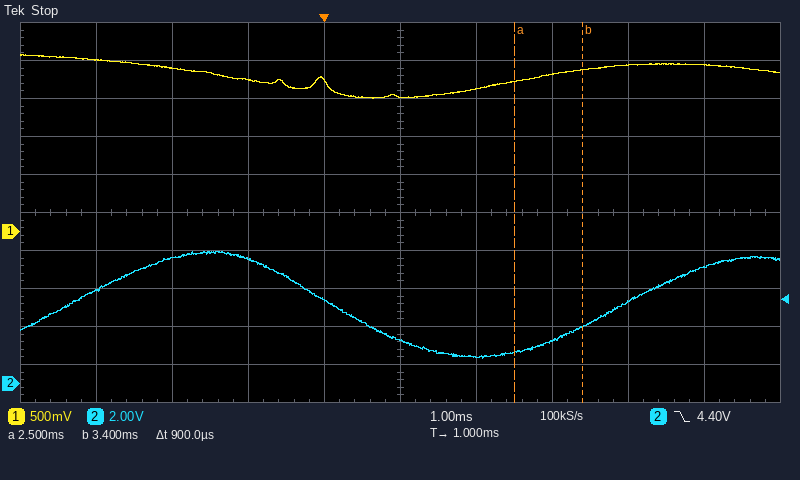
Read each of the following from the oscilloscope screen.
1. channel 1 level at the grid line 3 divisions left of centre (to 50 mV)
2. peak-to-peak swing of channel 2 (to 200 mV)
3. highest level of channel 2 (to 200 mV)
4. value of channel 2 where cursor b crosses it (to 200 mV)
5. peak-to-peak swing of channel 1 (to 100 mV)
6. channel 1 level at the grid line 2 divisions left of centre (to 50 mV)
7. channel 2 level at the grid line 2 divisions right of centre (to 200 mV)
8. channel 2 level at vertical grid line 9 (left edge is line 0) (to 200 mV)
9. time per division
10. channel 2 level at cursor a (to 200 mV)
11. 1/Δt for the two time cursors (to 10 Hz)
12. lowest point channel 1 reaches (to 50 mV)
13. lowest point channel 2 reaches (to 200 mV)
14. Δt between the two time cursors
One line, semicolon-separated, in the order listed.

2.15 V; 5.6 V; 7.0 V; 3.0 V; 600 mV; 2.00 V; 2.2 V; 6.2 V; 1 ms; 1.6 V; 1.11 kHz; 1.75 V; 1.4 V; 900 µs
